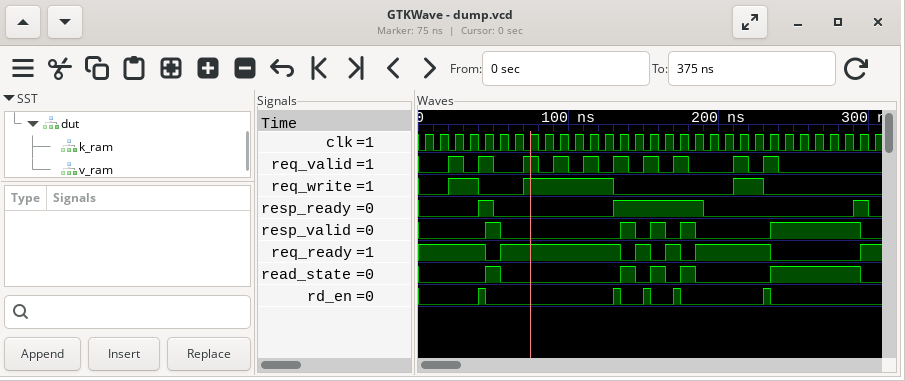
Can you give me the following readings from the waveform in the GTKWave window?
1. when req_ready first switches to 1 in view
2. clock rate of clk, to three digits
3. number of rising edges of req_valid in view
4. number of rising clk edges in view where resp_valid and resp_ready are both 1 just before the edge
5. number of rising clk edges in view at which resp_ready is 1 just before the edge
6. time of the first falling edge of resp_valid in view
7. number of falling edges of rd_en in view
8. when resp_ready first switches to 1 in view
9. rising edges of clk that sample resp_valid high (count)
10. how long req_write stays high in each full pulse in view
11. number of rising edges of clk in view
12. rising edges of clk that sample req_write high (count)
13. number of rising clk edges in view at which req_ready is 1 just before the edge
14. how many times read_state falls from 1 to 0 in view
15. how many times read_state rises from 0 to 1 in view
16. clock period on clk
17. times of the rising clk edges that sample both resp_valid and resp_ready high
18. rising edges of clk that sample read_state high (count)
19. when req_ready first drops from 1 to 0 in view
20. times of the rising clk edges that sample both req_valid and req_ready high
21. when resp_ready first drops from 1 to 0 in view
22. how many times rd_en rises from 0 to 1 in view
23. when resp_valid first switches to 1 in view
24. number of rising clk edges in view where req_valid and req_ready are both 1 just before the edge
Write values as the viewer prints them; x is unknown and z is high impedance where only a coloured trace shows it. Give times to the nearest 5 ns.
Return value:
55 ns
100 MHz
10
4
8
55 ns
5
40 ns
10
20 ns, 60 ns, 20 ns
31
10
21
5
5
10 ns
145 ns, 165 ns, 185 ns, 295 ns
10
45 ns
25 ns, 45 ns, 75 ns, 95 ns, 115 ns, 135 ns, 155 ns, 175 ns, 215 ns, 235 ns
50 ns
5
45 ns
10
